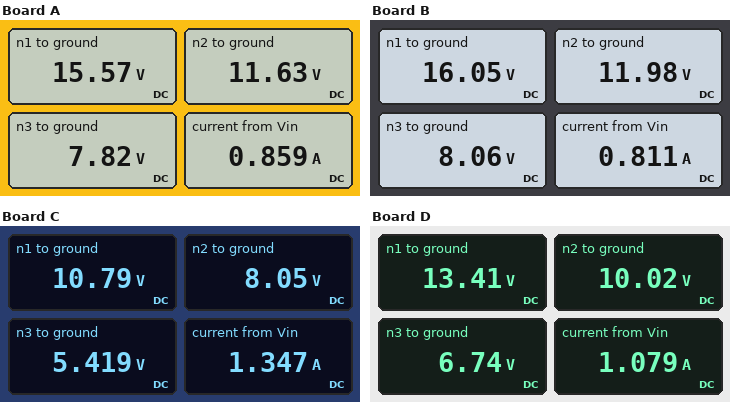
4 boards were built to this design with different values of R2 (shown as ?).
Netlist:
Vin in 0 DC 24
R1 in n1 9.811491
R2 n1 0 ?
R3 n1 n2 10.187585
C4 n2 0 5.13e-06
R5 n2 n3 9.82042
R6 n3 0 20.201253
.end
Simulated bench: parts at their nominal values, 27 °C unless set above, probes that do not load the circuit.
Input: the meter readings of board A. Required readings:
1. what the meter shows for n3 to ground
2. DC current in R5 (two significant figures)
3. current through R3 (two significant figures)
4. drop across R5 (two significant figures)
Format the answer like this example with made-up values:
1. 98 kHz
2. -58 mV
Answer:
1. 7.82 V
2. 390 mA
3. 390 mA
4. 3.8 V
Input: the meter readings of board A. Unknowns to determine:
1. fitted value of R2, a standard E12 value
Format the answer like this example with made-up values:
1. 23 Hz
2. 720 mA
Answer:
1. 33 Ω
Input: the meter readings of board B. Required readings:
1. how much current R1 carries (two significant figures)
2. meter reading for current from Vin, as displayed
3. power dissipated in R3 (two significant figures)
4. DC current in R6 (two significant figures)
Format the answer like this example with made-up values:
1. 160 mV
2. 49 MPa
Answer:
1. 810 mA
2. 0.811 A
3. 1.6 W
4. 400 mA
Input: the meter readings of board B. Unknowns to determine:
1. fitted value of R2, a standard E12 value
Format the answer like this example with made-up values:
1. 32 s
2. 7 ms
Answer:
1. 39 Ω
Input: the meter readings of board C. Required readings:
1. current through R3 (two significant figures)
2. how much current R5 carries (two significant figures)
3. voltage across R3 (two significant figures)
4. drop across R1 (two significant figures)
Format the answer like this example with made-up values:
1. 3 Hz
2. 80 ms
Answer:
1. 270 mA
2. 270 mA
3. 2.7 V
4. 13 V
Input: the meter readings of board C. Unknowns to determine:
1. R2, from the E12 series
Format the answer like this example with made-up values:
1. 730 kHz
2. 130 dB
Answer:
1. 10 Ω
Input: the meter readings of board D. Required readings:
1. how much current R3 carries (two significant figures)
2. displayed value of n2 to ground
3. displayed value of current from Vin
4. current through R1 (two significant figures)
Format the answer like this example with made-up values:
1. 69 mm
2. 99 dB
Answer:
1. 330 mA
2. 10.02 V
3. 1.079 A
4. 1.1 A
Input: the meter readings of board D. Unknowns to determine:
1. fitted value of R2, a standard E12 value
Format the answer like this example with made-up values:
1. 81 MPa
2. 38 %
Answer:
1. 18 Ω
